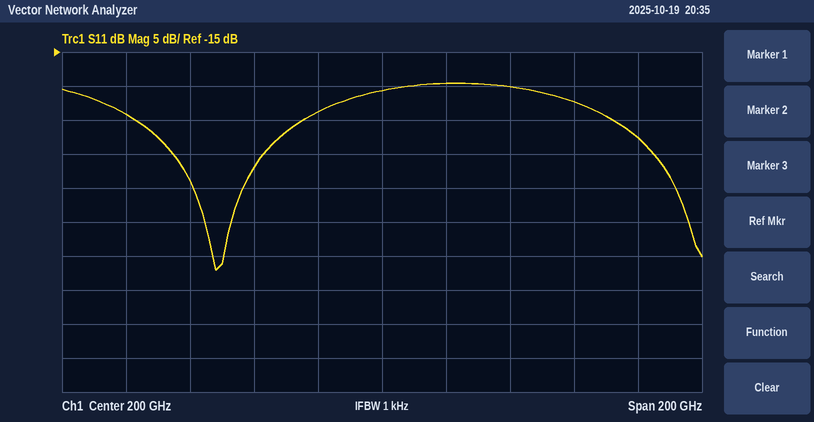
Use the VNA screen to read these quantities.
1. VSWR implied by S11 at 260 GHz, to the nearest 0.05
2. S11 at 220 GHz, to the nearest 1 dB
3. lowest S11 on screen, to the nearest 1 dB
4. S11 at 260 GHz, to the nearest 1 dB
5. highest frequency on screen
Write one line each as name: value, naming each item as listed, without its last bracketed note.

VSWR implied by S11 at 260 GHz, to the nearest 0.05: 1.15
S11 at 220 GHz, to the nearest 1 dB: -20 dB
lowest S11 on screen, to the nearest 1 dB: -47 dB
S11 at 260 GHz, to the nearest 1 dB: -22 dB
highest frequency on screen: 300 GHz
